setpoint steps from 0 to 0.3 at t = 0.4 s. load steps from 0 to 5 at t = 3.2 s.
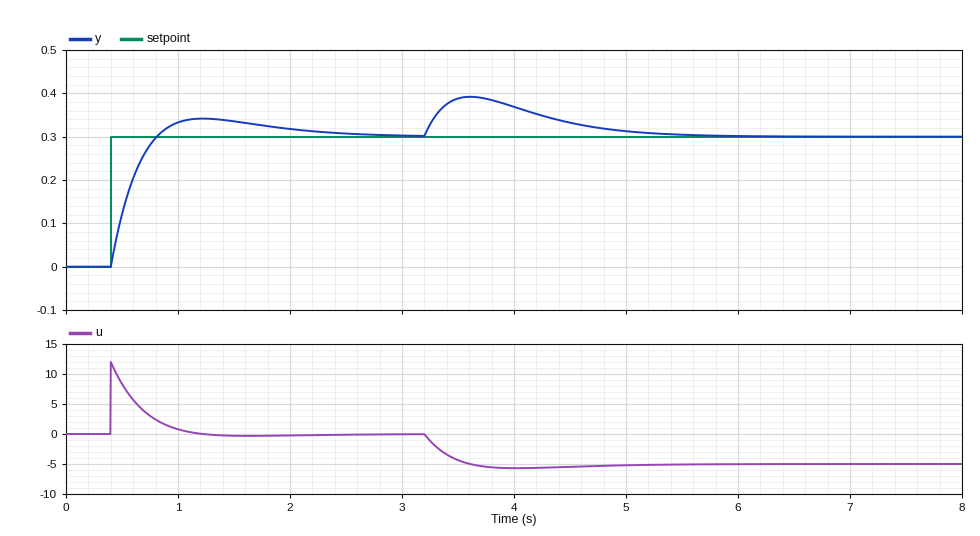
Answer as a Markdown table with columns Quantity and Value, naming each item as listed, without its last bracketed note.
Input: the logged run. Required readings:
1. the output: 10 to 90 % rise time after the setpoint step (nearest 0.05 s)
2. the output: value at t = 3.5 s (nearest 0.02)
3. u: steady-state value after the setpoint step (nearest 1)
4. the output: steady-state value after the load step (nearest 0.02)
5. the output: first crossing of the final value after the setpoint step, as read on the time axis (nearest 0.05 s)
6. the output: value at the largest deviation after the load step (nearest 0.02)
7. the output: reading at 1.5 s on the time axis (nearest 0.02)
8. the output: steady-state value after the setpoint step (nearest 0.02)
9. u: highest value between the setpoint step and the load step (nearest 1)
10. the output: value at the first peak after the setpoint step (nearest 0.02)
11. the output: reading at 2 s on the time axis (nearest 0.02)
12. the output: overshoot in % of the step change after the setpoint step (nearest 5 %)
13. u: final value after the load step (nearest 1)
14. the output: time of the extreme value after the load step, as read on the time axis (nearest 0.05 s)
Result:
| Quantity | Value |
|---|---|
| the output: 10 to 90 % rise time after the setpoint step | 0.30 s |
| the output: value at t = 3.5 s | 0.38 |
| u: steady-state value after the setpoint step | 0 |
| the output: steady-state value after the load step | 0.30 |
| the output: first crossing of the final value after the setpoint step, as read on the time axis | 0.80 s |
| the output: value at the largest deviation after the load step | 0.40 |
| the output: reading at 1.5 s on the time axis | 0.34 |
| the output: steady-state value after the setpoint step | 0.30 |
| u: highest value between the setpoint step and the load step | 12 |
| the output: value at the first peak after the setpoint step | 0.34 |
| the output: reading at 2 s on the time axis | 0.32 |
| the output: overshoot in % of the step change after the setpoint step | 15 % |
| u: final value after the load step | -5 |
| the output: time of the extreme value after the load step, as read on the time axis | 3.60 s |
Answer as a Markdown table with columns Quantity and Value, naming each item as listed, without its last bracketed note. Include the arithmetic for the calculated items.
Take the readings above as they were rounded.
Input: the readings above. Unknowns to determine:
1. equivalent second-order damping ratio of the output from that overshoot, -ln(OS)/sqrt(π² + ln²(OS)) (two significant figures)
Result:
| Quantity | Value |
|---|---|
| equivalent second-order damping ratio of the output from that overshoot, -ln(OS)/sqrt(π² + ln²(OS)) | ln(0.15) = -1.897; 1.897 / sqrt(9.870 + 3.599) = 0.52 |
